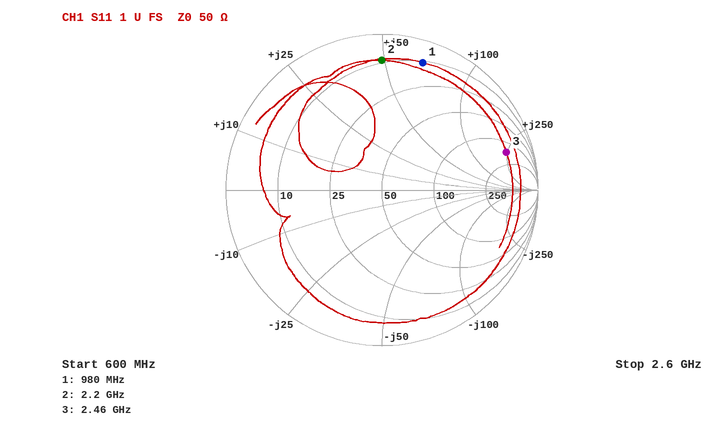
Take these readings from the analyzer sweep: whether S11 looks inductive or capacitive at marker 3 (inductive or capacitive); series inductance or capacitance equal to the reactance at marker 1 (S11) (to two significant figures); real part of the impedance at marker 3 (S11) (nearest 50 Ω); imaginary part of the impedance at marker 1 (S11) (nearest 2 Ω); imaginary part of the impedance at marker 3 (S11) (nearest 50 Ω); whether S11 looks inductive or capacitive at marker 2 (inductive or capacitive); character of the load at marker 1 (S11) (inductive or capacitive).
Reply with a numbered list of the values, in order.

1. inductive
2. 11 nH
3. 150 Ω
4. +68 Ω
5. +250 Ω
6. inductive
7. inductive
